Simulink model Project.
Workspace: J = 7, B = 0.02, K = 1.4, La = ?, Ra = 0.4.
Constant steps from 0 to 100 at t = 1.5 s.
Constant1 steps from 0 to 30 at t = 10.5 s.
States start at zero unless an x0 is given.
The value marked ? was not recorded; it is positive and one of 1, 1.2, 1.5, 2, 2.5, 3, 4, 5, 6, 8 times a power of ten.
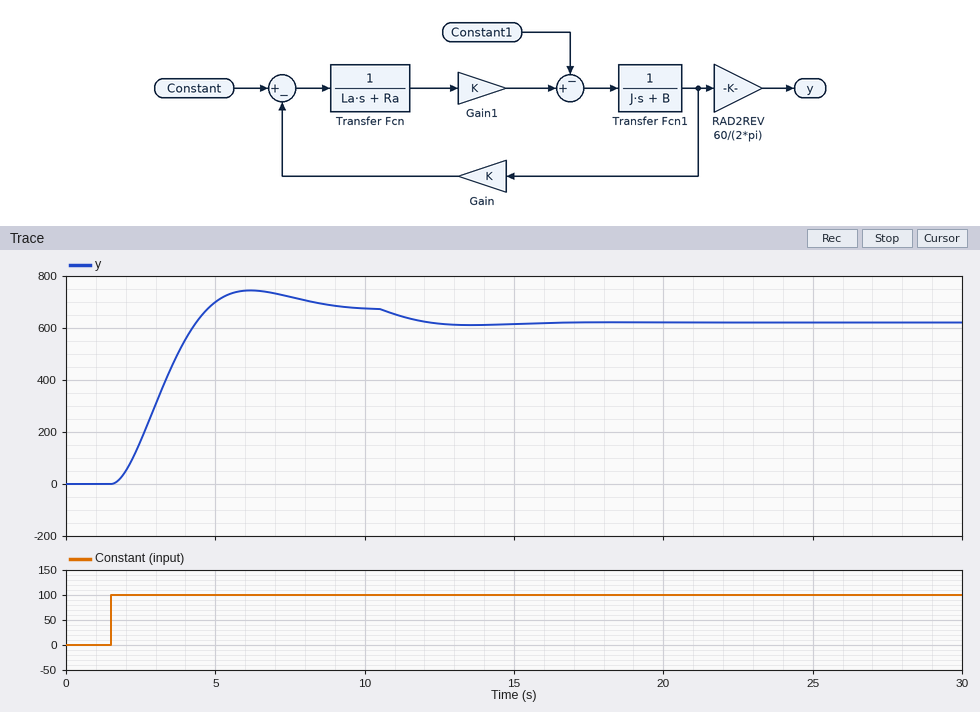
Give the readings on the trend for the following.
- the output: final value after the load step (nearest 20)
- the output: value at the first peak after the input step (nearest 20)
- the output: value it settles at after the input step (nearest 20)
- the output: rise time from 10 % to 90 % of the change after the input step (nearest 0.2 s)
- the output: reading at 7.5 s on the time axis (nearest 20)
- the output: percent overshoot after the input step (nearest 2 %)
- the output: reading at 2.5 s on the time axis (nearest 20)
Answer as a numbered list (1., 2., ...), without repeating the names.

1. 620
2. 740
3. 680
4. 2.2 s
5. 720
6. 10 %
7. 160
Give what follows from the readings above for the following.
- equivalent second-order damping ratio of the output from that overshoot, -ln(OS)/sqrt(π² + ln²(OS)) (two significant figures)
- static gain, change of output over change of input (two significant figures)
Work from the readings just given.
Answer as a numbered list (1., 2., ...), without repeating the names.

1. 0.59
2. 6.8
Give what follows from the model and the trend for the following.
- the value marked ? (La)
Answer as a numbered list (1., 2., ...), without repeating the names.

1. 0.4
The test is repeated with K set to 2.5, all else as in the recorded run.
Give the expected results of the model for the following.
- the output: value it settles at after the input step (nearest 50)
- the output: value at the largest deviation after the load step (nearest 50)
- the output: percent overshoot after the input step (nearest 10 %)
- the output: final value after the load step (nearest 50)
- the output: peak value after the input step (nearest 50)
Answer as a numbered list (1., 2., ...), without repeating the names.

1. 400
2. 350
3. 30 %
4. 350
5. 500
